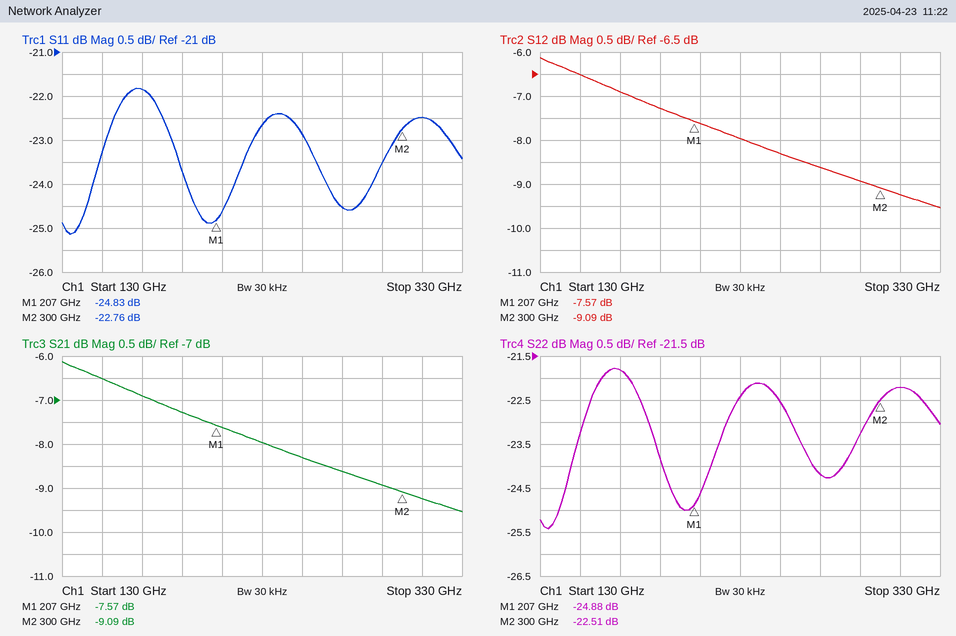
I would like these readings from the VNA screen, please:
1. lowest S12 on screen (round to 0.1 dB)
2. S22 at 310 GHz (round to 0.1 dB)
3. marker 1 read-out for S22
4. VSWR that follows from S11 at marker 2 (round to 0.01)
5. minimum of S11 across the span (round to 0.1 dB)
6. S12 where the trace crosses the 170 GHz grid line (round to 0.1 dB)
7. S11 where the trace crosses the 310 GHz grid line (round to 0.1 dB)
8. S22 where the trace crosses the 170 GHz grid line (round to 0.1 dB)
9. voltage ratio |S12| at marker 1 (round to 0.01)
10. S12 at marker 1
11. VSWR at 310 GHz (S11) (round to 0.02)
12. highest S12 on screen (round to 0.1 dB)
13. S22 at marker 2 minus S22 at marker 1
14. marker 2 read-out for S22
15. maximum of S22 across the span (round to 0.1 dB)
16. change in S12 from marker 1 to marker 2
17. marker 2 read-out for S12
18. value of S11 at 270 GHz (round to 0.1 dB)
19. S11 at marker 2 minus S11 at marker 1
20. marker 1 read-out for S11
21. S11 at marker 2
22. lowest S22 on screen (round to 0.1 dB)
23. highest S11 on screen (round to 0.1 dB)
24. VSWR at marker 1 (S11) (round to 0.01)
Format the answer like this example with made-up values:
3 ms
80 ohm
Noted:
-9.5 dB
-22.2 dB
-24.88 dB
1.16
-25.1 dB
-6.9 dB
-22.5 dB
-21.8 dB
0.42
-7.57 dB
1.16
-6.1 dB
2.37 dB
-22.51 dB
-21.8 dB
-1.52 dB
-9.09 dB
-24.5 dB
2.07 dB
-24.83 dB
-22.76 dB
-25.4 dB
-21.8 dB
1.12
